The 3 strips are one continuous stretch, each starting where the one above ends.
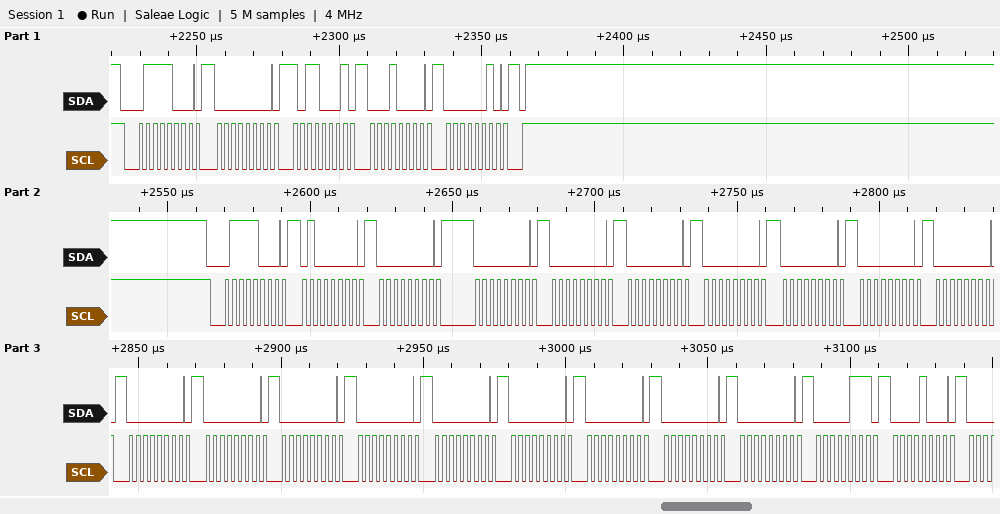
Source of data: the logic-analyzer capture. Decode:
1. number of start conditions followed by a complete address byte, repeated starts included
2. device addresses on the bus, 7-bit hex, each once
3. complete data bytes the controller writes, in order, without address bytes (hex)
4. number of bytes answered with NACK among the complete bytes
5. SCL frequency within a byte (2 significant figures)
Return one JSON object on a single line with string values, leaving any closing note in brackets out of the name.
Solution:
{"number of start conditions followed by a complete address byte, repeated starts included": "2", "device addresses on the bus, 7-bit hex, each once": "0x3C", "complete data bytes the controller writes, in order, without address bytes": "00 B1 10 02 40 00 00 00 00 00 00 00 00 00 00 00 00 00 00 00 00 00 07 08", "number of bytes answered with NACK among the complete bytes": "0", "SCL frequency within a byte": "400 kHz"}
